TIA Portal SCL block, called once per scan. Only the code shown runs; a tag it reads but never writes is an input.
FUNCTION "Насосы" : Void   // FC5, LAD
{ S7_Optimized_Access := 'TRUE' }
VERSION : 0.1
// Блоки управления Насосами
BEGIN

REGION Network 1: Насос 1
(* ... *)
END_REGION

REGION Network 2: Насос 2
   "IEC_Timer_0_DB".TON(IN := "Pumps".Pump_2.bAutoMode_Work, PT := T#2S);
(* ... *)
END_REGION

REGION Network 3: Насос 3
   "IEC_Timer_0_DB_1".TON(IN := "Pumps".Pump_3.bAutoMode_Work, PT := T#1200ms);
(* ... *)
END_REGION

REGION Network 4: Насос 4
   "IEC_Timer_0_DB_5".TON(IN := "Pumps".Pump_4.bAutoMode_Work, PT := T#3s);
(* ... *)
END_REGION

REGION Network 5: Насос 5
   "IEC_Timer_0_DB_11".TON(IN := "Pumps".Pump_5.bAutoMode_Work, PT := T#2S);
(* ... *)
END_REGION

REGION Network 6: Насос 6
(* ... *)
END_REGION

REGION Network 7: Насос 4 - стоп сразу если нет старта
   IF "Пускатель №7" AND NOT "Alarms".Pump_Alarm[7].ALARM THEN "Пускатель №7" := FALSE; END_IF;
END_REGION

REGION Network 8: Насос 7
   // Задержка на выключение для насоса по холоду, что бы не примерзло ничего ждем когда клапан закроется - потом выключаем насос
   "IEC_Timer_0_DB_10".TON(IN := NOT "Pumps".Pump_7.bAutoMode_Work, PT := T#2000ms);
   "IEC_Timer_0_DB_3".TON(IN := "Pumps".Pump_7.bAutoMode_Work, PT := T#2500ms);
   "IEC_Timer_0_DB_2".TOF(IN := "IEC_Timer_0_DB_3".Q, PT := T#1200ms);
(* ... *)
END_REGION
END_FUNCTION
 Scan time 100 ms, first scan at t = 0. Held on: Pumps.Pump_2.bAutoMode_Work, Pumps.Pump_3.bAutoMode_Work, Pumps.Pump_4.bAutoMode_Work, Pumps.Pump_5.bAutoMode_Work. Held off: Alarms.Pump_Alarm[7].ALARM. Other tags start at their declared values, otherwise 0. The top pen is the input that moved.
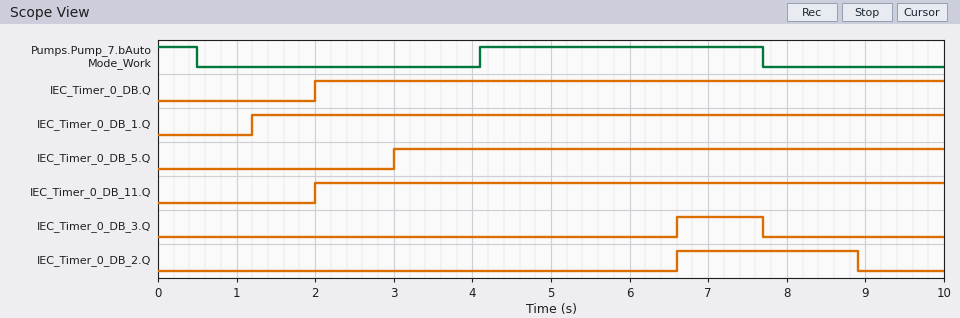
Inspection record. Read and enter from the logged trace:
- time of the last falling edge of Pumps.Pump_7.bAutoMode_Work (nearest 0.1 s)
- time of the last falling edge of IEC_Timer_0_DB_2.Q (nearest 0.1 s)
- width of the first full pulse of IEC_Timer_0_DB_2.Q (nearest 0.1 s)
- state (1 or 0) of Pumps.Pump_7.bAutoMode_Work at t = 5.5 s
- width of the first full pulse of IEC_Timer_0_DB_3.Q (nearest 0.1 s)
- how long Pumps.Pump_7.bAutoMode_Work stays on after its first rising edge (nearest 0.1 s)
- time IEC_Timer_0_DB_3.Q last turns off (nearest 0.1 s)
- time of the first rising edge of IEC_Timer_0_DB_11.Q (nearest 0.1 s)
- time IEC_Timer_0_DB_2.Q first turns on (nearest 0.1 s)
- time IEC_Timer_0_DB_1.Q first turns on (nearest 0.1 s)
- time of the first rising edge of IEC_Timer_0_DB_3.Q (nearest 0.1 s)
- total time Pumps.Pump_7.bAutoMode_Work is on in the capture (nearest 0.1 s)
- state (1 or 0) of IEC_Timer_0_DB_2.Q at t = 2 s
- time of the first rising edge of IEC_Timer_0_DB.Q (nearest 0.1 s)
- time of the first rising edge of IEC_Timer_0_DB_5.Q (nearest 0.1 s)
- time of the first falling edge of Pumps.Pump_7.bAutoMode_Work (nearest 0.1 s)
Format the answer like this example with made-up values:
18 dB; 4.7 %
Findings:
7.7 s; 8.9 s; 2.3 s; 1; 1.1 s; 3.6 s; 7.7 s; 2.0 s; 6.6 s; 1.2 s; 6.6 s; 4.1 s; 0; 2.0 s; 3.0 s; 0.5 s
